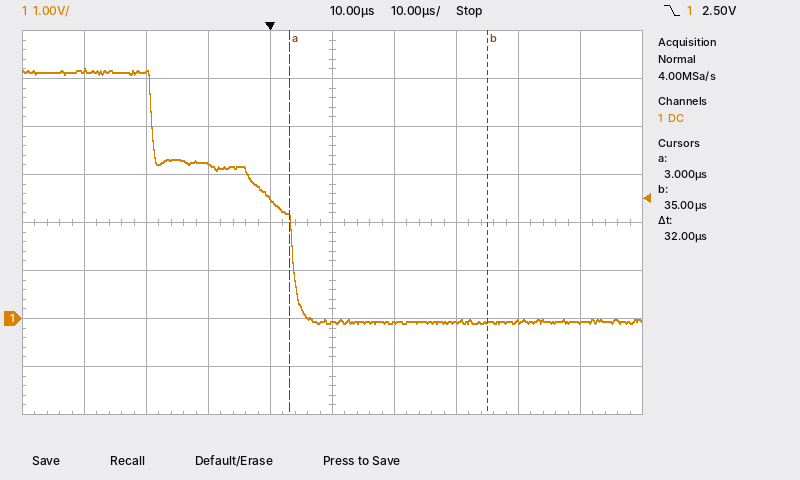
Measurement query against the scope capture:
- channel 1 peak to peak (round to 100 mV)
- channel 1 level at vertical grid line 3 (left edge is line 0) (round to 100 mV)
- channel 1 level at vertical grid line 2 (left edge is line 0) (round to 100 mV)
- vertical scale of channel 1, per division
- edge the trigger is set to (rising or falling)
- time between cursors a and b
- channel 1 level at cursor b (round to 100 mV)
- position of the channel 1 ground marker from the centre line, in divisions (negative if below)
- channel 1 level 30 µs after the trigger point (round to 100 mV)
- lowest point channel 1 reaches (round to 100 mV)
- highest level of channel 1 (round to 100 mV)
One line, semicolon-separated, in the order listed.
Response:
5.3 V; 3.2 V; 5.1 V; 1 V; falling; 32 µs; -100 mV; -2.0 div; -100 mV; -100 mV; 5.2 V
